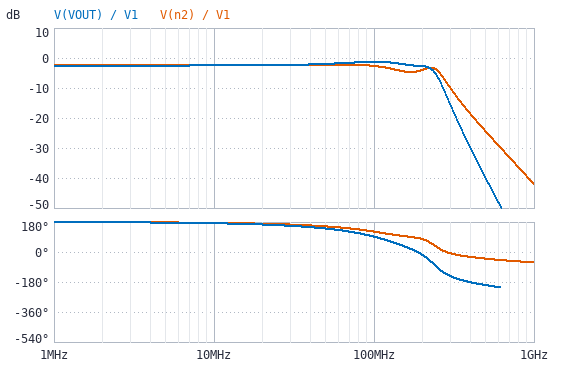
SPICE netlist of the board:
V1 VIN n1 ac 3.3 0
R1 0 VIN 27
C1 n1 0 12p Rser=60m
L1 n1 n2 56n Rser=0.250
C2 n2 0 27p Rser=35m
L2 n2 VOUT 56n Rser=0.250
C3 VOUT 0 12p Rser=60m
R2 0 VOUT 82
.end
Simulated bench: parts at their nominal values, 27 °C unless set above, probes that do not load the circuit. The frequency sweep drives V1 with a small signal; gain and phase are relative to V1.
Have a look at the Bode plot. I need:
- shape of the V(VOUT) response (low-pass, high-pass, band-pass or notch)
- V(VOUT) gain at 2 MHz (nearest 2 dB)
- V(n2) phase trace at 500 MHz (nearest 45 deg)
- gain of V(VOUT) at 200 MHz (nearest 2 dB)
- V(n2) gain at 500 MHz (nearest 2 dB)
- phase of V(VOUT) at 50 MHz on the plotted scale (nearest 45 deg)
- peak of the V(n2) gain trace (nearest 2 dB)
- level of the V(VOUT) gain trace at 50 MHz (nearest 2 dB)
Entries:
low-pass
-2 dB
-45 deg
-2 dB
-24 dB
135 deg
-2 dB
-2 dB
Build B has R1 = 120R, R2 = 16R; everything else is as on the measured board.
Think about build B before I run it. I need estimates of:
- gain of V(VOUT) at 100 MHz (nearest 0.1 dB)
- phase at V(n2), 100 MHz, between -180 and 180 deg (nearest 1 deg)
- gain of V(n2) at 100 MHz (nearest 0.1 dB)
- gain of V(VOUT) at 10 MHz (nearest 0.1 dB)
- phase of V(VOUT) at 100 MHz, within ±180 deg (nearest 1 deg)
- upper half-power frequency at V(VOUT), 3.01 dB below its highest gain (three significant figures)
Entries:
-14.9 dB
164 deg
-7.6 dB
-18.6 dB
93 deg
161 MHz
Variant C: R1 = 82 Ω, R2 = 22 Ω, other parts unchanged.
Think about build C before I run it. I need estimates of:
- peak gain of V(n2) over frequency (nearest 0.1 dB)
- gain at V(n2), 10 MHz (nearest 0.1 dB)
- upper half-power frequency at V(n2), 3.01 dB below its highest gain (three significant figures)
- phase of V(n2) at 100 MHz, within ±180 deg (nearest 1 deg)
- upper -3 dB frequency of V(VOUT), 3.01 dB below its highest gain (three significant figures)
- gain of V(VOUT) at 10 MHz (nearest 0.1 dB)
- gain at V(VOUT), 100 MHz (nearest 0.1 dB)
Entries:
-3.3 dB
-13.3 dB
256 MHz
157 deg
230 MHz
-13.5 dB
-11.9 dB
